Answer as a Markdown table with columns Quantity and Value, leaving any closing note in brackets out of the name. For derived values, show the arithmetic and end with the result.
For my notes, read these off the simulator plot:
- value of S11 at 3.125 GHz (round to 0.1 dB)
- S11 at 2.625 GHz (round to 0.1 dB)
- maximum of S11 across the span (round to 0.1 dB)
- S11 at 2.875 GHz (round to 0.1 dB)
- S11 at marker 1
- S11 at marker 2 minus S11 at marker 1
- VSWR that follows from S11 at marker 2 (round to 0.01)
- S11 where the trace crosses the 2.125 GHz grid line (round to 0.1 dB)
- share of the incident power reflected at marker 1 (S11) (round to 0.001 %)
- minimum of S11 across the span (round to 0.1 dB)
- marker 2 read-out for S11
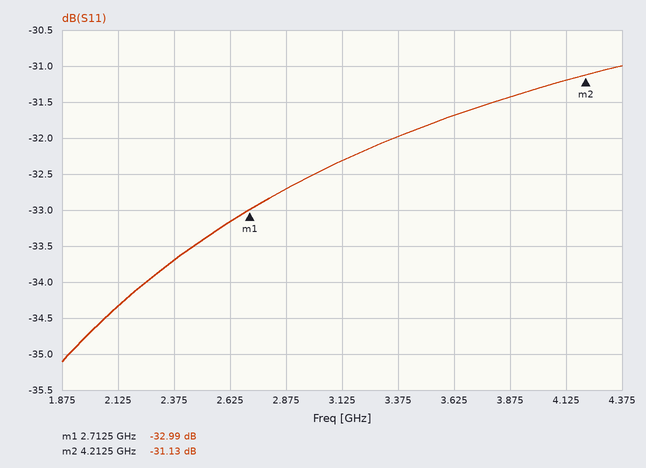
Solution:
| Quantity | Value |
|---|---|
| value of S11 at 3.125 GHz | -32.3 dB |
| S11 at 2.625 GHz | -33.2 dB |
| maximum of S11 across the span | -31.0 dB |
| S11 at 2.875 GHz | -32.7 dB |
| S11 at marker 1 | -32.99 dB |
| S11 at marker 2 minus S11 at marker 1 | -31.13 − (-32.99) = 1.86 dB |
| VSWR that follows from S11 at marker 2 | (1 + 0.0278)/(1 − 0.0278) ≈ 1.06 |
| S11 where the trace crosses the 2.125 GHz grid line | -34.3 dB |
| share of the incident power reflected at marker 1 (S11) | 10^(-32.99/10) ≈ 0.050 % |
| minimum of S11 across the span | -35.1 dB |
| marker 2 read-out for S11 | -31.13 dB |
